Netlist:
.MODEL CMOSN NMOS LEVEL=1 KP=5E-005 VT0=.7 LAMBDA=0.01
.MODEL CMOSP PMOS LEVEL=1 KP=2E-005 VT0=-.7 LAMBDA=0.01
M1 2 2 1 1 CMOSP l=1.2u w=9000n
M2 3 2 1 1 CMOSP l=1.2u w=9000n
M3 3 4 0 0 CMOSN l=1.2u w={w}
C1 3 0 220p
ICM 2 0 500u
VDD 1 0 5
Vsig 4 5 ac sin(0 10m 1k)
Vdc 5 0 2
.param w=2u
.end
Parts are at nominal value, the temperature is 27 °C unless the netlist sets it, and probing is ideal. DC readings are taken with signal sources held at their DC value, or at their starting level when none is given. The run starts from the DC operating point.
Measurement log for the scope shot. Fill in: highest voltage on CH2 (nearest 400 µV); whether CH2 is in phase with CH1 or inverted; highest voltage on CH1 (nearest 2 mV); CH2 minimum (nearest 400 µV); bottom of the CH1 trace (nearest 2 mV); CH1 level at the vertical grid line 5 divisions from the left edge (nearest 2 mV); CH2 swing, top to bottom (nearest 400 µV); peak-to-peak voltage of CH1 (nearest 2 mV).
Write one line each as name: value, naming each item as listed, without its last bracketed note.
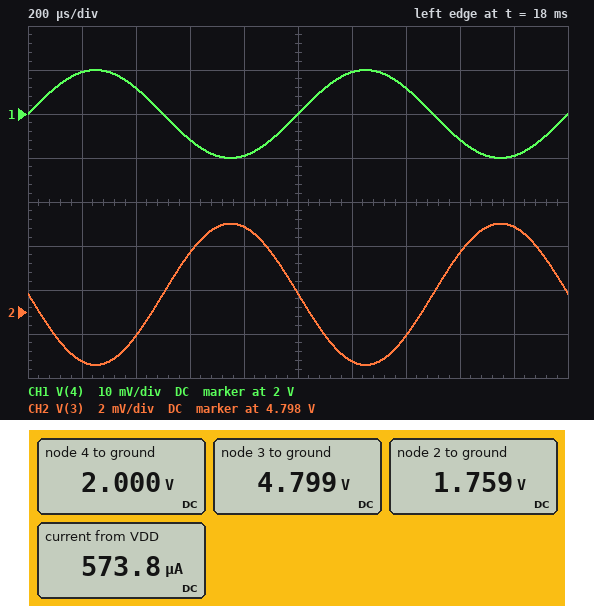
highest voltage on CH2: 4.8020 V
whether CH2 is in phase with CH1 or inverted: inverted
highest voltage on CH1: 2.010 V
CH2 minimum: 4.7956 V
bottom of the CH1 trace: 1.990 V
CH1 level at the vertical grid line 5 divisions from the left edge: 2.000 V
CH2 swing, top to bottom: 6.4 mV
peak-to-peak voltage of CH1: 20 mV
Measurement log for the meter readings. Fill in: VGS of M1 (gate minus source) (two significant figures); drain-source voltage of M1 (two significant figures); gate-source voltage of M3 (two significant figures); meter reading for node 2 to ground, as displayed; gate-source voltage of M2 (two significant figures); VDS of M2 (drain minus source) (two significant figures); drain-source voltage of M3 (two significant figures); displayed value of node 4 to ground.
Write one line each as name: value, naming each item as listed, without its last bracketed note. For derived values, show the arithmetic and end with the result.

VGS of M1 (gate minus source): 1.759 V - 5 V = -3.2 V
drain-source voltage of M1: 1.759 V - 5 V = -3.2 V
gate-source voltage of M3: 2 V = 2.0 V
meter reading for node 2 to ground, as displayed: 1.759 V
gate-source voltage of M2: 1.759 V - 5 V = -3.2 V
VDS of M2 (drain minus source): 4.799 V - 5 V = -200 mV
drain-source voltage of M3: 4.799 V = 4.8 V
displayed value of node 4 to ground: 2.000 V
